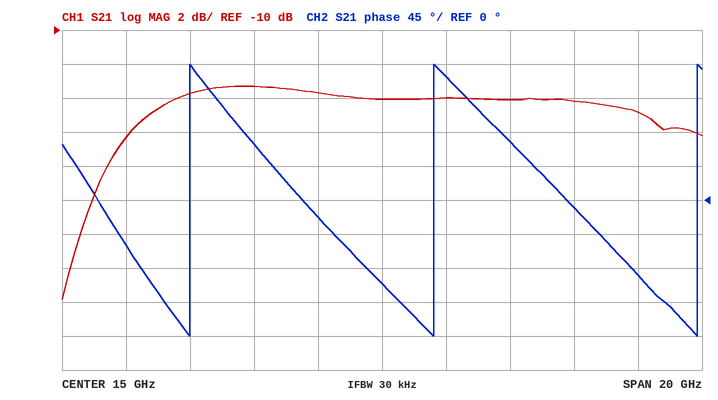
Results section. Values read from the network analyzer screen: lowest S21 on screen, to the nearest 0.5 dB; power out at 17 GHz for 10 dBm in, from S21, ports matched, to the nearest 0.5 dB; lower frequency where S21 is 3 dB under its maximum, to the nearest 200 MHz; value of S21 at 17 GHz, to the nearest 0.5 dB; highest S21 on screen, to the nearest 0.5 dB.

-26.0 dB
-4.0 dBm
7.0 GHz
-14.0 dB
-13.5 dB
